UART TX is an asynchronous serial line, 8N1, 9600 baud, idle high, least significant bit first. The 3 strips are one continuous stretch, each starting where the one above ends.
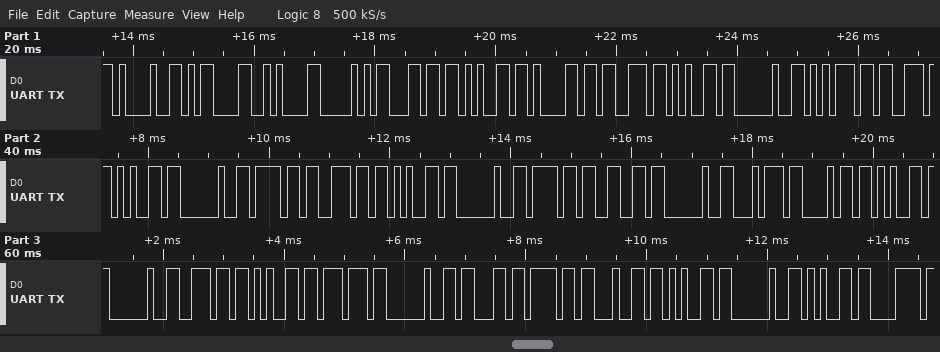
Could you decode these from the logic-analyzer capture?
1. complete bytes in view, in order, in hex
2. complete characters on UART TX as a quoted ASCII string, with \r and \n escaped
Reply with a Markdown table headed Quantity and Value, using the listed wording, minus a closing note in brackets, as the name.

| Quantity | Value |
|---|---|
| complete bytes in view, in order, in hex | 0x21 0x0D 0x0A 0x50 0x6C 0x65 0x61 0x73 0x65 0x20 0x75 0x73 0x65 0x20 0x6F 0x6E 0x65 0x20 0x6F 0x66 0x20 0x74 0x68 0x65 0x20 0x6E 0x65 0x77 0x20 0x63 0x6F 0x64 0x65 0x20 0x65 0x78 |
| complete characters on UART TX as a quoted ASCII string, with \r and \n escaped | "!\r\nPlease use one of the new code ex" |
